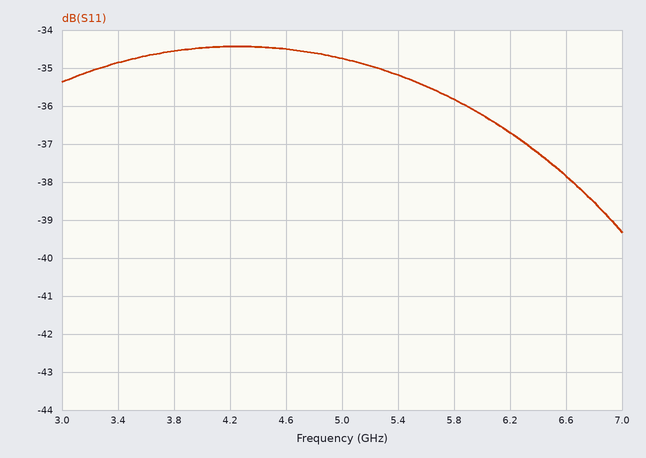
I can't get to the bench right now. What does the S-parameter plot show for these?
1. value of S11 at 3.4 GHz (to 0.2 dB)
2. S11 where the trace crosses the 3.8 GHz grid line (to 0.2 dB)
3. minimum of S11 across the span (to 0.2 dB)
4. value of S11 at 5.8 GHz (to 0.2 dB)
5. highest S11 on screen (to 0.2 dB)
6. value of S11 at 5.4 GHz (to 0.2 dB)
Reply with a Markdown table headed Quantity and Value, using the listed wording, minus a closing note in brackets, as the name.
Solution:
| Quantity | Value |
|---|---|
| value of S11 at 3.4 GHz | -34.8 dB |
| S11 where the trace crosses the 3.8 GHz grid line | -34.6 dB |
| minimum of S11 across the span | -39.4 dB |
| value of S11 at 5.8 GHz | -35.8 dB |
| highest S11 on screen | -34.4 dB |
| value of S11 at 5.4 GHz | -35.2 dB |
